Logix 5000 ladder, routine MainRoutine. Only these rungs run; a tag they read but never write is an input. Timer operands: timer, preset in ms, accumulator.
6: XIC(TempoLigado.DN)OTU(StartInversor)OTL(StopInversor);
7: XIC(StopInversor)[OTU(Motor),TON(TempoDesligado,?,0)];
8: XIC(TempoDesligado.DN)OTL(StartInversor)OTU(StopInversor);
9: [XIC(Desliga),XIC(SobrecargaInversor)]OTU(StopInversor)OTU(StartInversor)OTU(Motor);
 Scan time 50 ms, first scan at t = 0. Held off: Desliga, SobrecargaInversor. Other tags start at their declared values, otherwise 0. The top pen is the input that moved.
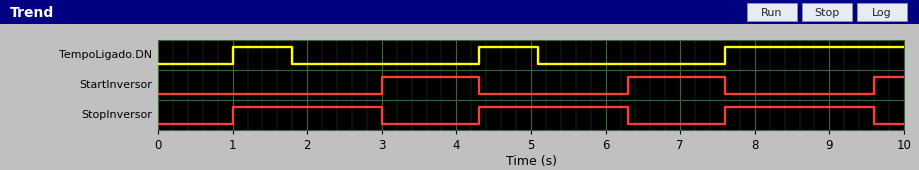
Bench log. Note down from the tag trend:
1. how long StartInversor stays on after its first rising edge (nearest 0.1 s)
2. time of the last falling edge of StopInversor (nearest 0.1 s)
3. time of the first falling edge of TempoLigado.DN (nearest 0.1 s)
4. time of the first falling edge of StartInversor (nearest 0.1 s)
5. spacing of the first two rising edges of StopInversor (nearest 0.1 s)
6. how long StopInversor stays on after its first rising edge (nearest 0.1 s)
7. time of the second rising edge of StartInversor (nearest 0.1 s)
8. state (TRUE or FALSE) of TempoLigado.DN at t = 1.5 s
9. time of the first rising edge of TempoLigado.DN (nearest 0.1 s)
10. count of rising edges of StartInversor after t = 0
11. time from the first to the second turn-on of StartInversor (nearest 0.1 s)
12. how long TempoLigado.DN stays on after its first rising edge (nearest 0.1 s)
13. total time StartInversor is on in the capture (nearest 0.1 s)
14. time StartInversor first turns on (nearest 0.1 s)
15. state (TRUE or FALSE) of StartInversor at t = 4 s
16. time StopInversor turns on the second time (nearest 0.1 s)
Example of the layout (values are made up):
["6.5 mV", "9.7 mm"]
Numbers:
["1.3 s", "9.6 s", "1.8 s", "4.3 s", "3.3 s", "2.0 s", "6.3 s", "TRUE", "1.0 s", "3", "3.3 s", "0.8 s", "3.0 s", "3.0 s", "TRUE", "4.3 s"]
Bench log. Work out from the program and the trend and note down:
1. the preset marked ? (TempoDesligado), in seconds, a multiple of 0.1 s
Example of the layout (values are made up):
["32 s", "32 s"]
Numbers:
["2.0 s"]
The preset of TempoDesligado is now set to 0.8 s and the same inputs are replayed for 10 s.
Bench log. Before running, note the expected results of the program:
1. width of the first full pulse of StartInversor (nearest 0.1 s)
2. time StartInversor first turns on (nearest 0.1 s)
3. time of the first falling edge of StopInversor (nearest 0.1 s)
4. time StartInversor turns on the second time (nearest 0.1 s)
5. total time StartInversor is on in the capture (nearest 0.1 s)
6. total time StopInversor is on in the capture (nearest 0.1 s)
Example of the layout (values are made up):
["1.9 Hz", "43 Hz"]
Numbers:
["2.5 s", "1.8 s", "1.8 s", "5.1 s", "6.6 s", "2.4 s"]
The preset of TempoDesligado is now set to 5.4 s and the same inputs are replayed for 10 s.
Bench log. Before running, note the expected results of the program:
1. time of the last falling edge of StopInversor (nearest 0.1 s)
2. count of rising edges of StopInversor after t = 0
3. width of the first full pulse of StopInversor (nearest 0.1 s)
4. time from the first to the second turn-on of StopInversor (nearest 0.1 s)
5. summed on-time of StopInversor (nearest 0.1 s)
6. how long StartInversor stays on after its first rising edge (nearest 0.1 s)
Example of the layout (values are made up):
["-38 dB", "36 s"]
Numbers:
["6.4 s", "2", "5.4 s", "6.6 s", "7.8 s", "1.2 s"]
